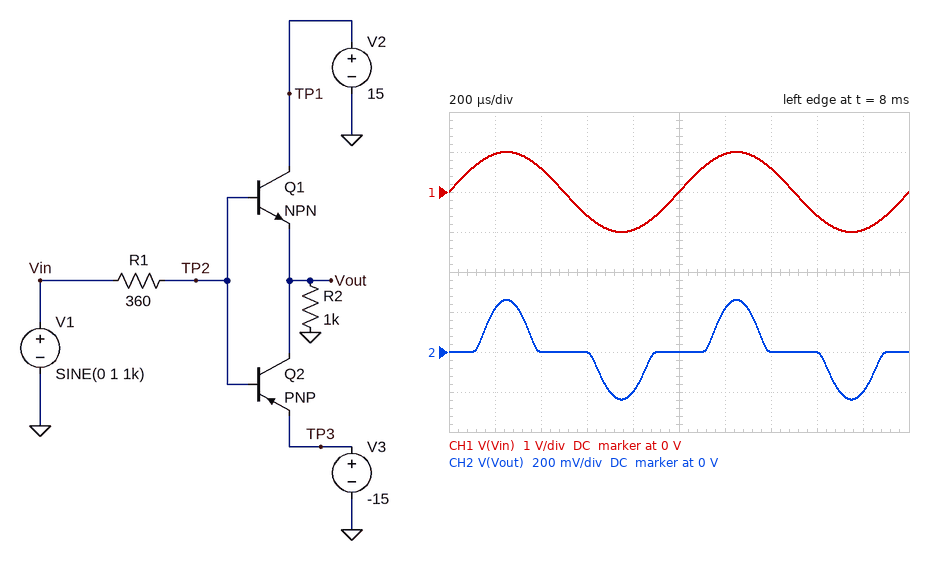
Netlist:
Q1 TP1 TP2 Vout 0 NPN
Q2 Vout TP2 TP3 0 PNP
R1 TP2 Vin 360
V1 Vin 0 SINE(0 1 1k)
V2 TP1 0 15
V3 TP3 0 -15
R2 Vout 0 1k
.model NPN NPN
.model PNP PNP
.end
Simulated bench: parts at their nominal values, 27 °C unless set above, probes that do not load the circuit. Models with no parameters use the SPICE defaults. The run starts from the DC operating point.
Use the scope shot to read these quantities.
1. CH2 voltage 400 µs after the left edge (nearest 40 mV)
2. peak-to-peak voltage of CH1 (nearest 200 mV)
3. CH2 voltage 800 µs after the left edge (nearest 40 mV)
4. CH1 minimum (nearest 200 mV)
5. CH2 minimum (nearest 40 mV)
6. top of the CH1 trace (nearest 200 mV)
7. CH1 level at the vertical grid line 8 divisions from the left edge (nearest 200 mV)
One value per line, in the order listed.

0 V
2.0 V
-200 mV
-1.0 V
-240 mV
1.0 V
-600 mV
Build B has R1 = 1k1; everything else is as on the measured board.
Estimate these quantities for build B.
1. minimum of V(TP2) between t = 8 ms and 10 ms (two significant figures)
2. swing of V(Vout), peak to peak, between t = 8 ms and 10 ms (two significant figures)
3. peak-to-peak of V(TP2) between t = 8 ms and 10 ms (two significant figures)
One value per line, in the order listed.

-900 mV
440 mV
1.9 V
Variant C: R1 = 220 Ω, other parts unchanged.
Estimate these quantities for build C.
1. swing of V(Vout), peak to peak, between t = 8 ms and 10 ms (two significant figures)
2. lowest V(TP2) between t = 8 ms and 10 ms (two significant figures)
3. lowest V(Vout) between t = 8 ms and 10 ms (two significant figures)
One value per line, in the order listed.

510 mV
-970 mV
-250 mV
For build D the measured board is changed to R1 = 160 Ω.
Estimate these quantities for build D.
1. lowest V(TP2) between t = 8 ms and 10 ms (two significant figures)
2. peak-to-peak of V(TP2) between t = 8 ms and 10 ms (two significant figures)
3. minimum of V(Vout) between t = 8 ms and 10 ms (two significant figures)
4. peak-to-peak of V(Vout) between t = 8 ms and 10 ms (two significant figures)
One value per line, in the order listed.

-980 mV
2.0 V
-260 mV
520 mV
